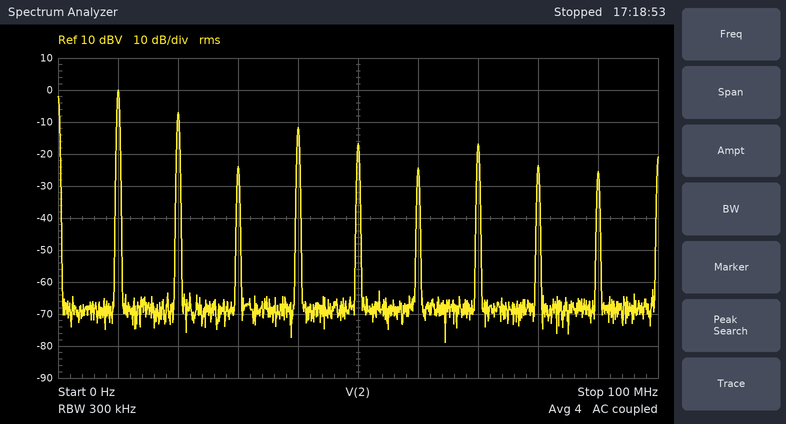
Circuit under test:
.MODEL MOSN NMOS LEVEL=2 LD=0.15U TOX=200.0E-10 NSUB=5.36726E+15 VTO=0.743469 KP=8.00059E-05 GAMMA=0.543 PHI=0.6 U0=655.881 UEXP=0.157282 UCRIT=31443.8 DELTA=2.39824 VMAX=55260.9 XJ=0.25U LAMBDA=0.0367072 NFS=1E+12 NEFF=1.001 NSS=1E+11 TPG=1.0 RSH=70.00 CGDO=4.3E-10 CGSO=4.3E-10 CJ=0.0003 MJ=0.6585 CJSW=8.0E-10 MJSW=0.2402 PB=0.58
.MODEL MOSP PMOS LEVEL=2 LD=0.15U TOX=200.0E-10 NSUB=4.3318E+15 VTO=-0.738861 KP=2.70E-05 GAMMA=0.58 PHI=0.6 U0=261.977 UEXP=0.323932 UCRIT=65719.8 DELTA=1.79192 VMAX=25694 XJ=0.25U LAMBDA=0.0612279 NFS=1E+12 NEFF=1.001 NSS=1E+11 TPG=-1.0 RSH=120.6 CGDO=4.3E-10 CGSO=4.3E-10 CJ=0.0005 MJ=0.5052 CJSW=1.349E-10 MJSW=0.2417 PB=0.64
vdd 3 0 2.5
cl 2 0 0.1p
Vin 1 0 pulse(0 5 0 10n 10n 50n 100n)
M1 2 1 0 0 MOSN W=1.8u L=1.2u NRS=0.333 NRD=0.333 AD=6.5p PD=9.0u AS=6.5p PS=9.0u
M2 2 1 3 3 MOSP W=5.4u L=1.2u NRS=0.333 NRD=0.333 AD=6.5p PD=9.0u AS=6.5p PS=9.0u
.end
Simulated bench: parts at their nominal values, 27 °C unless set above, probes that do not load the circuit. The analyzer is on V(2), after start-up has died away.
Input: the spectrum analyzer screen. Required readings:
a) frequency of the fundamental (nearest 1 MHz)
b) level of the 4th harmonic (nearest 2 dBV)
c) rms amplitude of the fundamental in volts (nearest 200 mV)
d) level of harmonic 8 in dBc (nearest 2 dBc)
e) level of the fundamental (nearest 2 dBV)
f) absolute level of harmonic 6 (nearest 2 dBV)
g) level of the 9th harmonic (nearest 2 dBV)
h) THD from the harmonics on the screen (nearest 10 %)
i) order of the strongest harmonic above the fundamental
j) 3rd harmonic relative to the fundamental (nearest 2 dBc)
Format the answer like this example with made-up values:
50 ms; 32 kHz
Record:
10 MHz; -12 dBV; 1.0 V; -24 dBc; 0 dBV; -24 dBV; -26 dBV; 60 %; 2; -24 dBc
